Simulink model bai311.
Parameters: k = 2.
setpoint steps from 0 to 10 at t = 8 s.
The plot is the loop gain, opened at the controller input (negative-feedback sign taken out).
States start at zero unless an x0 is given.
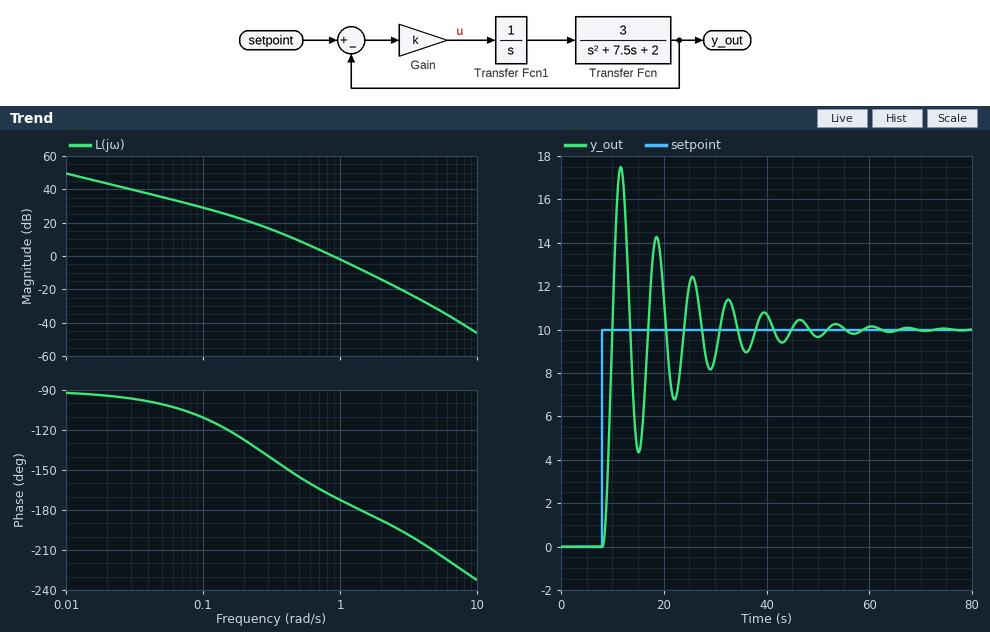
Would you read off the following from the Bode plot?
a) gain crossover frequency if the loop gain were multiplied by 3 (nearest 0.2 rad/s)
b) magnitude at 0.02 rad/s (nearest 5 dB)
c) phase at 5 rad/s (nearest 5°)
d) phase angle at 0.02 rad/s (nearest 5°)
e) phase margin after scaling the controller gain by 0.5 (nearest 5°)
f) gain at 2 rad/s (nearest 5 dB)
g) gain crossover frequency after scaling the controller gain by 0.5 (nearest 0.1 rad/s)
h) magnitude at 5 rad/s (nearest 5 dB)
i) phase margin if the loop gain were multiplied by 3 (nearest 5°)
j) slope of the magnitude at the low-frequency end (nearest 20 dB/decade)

1.6 rad/s
45 dB
-210°
-95°
20°
-15 dB
0.6 rad/s
-30 dB
0°
-20 dB/decade
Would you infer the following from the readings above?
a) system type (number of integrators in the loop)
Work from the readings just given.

1
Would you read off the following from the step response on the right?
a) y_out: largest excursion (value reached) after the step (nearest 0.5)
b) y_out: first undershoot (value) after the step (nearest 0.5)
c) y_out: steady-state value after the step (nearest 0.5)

17.5
4.5
10.0
